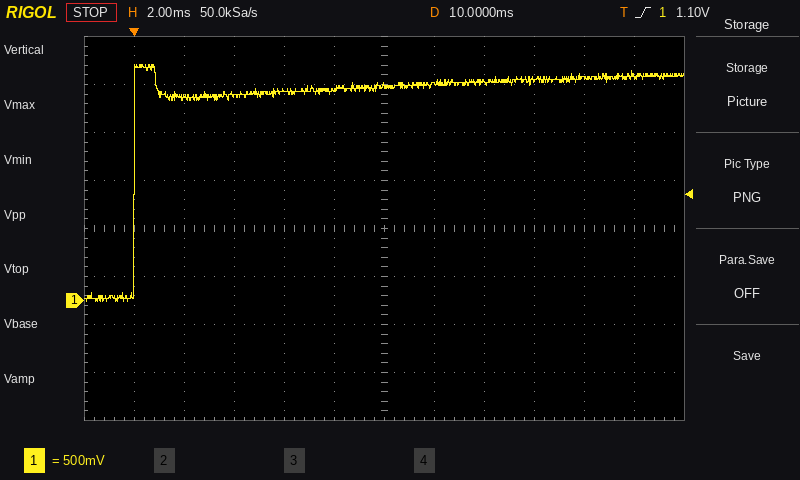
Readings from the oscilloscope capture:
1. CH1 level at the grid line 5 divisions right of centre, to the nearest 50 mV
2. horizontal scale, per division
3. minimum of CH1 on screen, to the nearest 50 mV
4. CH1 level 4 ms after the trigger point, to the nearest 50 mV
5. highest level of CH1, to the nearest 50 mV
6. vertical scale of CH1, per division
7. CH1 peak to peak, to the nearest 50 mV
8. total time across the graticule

2.35 V
2 ms
0 mV
2.15 V
2.45 V
500 mV
2.45 V
24 ms
